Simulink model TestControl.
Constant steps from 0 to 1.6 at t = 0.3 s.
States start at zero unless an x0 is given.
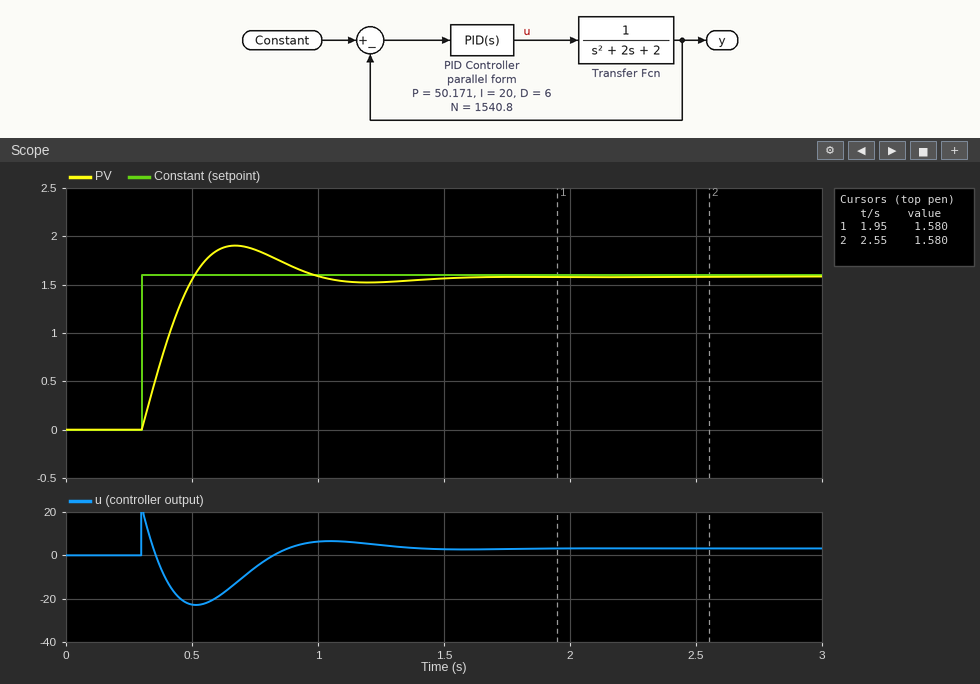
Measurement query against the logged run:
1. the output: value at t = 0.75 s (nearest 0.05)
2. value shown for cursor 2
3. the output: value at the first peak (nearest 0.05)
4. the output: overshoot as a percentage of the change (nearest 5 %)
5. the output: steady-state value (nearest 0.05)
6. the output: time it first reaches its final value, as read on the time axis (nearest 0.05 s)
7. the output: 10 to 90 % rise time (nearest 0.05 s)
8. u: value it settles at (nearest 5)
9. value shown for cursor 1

1.85
1.580
1.90
20 %
1.60
0.50 s
0.15 s
5
1.580
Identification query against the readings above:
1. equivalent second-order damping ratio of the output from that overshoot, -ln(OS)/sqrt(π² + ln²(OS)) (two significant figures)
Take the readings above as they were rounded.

0.46
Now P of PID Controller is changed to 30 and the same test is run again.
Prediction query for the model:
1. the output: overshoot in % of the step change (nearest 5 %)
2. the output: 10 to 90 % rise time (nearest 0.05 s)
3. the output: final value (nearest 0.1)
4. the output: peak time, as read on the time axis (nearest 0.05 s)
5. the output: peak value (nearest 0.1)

10 %
0.20 s
1.6
0.80 s
1.8
